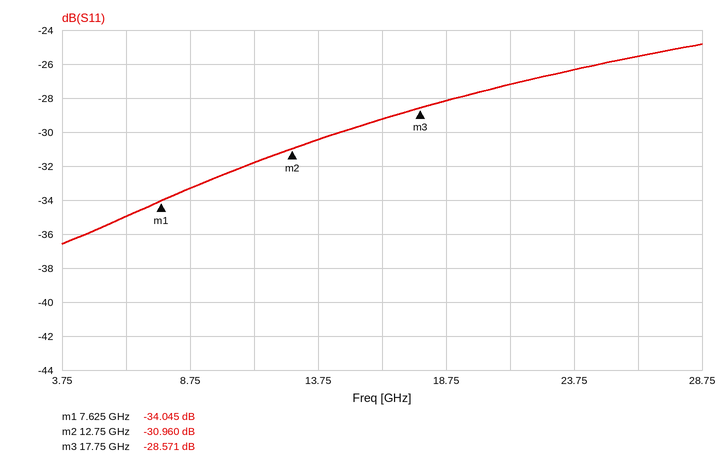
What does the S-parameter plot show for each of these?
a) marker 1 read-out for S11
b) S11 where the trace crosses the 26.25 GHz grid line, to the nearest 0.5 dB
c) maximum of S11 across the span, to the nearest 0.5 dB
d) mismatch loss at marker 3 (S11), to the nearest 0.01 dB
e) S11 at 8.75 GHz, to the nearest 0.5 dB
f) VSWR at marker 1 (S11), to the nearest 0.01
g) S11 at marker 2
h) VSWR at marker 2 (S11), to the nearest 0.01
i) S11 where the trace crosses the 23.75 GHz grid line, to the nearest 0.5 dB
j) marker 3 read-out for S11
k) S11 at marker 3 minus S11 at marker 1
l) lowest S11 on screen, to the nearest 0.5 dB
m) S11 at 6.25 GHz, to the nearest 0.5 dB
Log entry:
-34.045 dB
-25.5 dB
-25.0 dB
0.01 dB
-33.5 dB
1.04
-30.960 dB
1.06
-26.5 dB
-28.571 dB
5.474 dB
-36.5 dB
-35.0 dB
